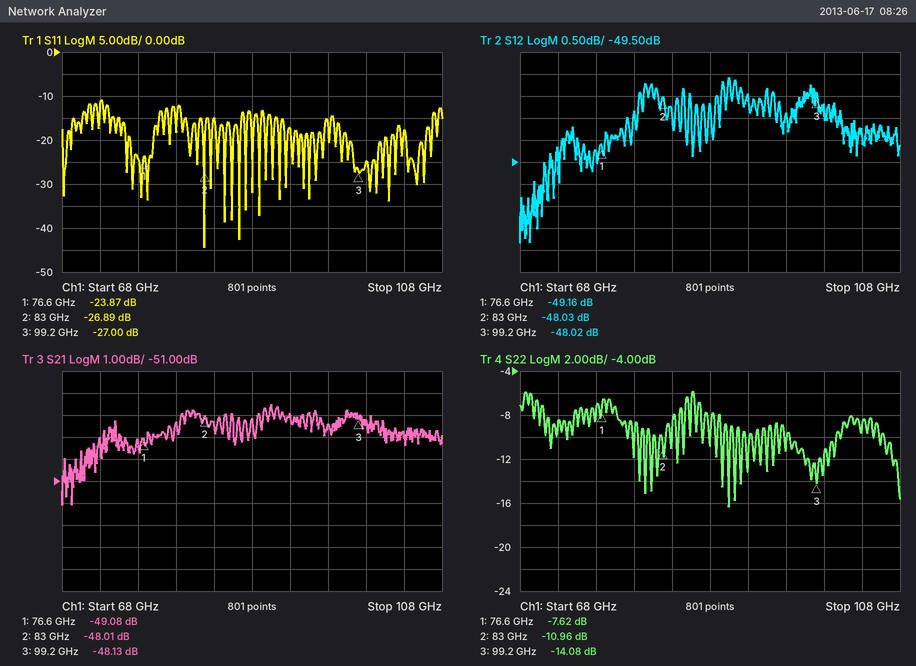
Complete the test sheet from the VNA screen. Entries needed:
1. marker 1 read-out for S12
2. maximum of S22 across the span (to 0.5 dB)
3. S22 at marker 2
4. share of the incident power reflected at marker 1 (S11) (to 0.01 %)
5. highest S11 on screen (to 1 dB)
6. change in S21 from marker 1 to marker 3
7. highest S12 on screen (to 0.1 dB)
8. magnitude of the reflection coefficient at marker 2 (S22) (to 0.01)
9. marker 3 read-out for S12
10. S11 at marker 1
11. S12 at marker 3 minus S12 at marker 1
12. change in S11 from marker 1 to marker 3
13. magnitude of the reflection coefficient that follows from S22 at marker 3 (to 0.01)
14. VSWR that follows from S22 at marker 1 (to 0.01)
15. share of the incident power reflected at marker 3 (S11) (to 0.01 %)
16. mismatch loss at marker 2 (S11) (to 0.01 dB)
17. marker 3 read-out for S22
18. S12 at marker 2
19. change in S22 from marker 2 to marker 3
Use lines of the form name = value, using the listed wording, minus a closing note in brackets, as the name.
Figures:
marker 1 read-out for S12 = -49.16 dB
maximum of S22 across the span = -6.0 dB
S22 at marker 2 = -10.96 dB
share of the incident power reflected at marker 1 (S11) = 0.41 %
highest S11 on screen = -11 dB
change in S21 from marker 1 to marker 3 = 0.95 dB
highest S12 on screen = -47.6 dB
magnitude of the reflection coefficient at marker 2 (S22) = 0.28
marker 3 read-out for S12 = -48.02 dB
S11 at marker 1 = -23.87 dB
S12 at marker 3 minus S12 at marker 1 = 1.14 dB
change in S11 from marker 1 to marker 3 = -3.13 dB
magnitude of the reflection coefficient that follows from S22 at marker 3 = 0.20
VSWR that follows from S22 at marker 1 = 2.42
share of the incident power reflected at marker 3 (S11) = 0.20 %
mismatch loss at marker 2 (S11) = 0.01 dB
marker 3 read-out for S22 = -14.08 dB
S12 at marker 2 = -48.03 dB
change in S22 from marker 2 to marker 3 = -3.12 dB
